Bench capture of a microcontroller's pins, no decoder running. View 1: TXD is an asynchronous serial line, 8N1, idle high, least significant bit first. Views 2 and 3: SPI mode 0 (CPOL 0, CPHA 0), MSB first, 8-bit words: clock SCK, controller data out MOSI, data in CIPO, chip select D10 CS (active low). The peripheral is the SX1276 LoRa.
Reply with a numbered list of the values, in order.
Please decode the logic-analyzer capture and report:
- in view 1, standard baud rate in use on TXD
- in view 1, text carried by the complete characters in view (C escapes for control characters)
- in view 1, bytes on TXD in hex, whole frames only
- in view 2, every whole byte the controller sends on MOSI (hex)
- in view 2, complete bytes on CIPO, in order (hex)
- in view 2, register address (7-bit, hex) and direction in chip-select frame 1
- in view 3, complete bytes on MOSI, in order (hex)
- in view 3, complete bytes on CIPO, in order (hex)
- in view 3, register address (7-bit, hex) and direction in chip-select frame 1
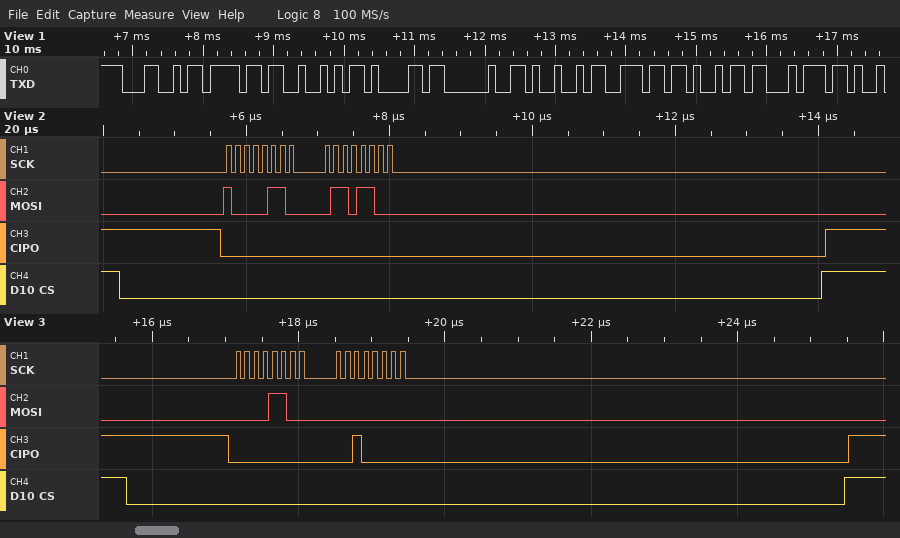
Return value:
1. 9600 baud
2. "LoRa Init"
3. 0x4C 0x6F 0x52 0x61 0x20 0x49 0x6E 0x69 0x74
4. 0x86 0x6C
5. 0x00 0x00
6. 0x06 write
7. 0C 00
8. 00 20
9. 0x0C read
